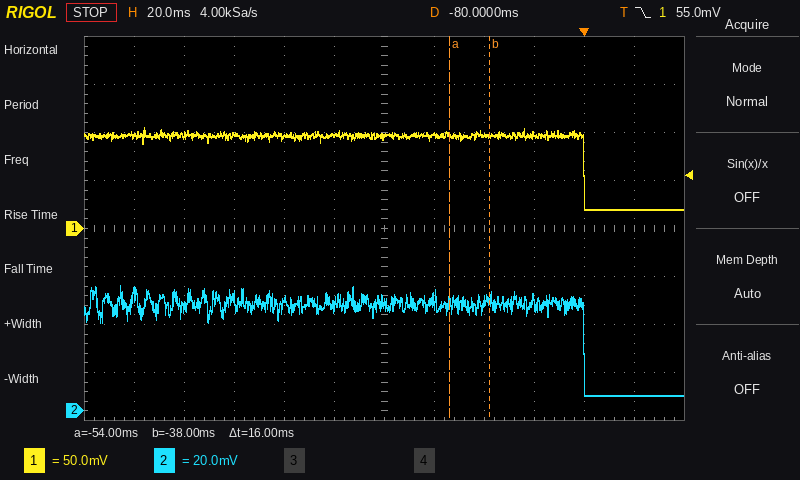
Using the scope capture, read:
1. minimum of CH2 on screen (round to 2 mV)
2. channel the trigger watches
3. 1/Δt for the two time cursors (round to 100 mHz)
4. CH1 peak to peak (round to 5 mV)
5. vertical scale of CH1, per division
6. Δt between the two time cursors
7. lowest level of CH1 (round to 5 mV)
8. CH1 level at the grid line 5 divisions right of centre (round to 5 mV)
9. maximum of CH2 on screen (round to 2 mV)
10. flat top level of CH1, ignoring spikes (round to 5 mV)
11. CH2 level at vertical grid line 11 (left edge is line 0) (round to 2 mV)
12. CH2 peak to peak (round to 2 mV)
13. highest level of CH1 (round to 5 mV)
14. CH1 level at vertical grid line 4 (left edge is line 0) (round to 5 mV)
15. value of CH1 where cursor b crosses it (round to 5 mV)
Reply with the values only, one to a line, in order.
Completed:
6 mV
CH1
62.5 Hz
85 mV
50 mV
16 ms
20 mV
20 mV
52 mV
95 mV
6 mV
46 mV
105 mV
95 mV
95 mV
